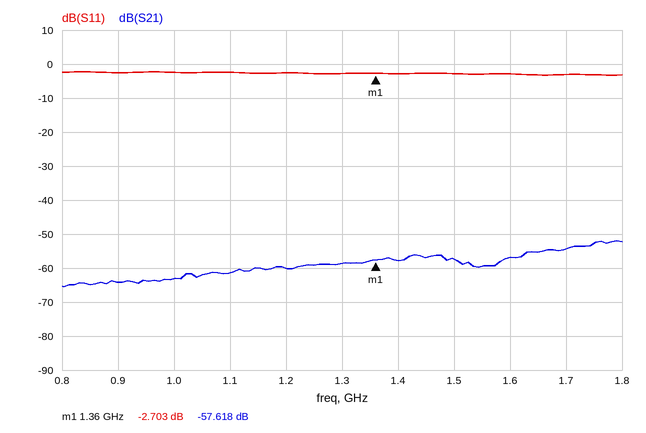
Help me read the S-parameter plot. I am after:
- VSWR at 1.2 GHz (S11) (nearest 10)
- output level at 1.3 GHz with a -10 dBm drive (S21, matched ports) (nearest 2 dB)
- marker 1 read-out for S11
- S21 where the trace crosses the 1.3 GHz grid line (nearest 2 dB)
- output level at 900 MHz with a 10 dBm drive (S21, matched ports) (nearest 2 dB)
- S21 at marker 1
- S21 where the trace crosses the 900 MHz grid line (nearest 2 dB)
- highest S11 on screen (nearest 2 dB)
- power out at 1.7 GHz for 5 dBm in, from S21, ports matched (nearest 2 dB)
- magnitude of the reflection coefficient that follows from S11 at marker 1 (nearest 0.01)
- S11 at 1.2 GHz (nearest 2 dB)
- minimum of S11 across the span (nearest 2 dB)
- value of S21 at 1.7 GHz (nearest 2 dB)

10
-68 dBm
-2.703 dB
-58 dB
-54 dBm
-57.618 dB
-64 dB
-2 dB
-50 dBm
0.73
-2 dB
-4 dB
-54 dB
